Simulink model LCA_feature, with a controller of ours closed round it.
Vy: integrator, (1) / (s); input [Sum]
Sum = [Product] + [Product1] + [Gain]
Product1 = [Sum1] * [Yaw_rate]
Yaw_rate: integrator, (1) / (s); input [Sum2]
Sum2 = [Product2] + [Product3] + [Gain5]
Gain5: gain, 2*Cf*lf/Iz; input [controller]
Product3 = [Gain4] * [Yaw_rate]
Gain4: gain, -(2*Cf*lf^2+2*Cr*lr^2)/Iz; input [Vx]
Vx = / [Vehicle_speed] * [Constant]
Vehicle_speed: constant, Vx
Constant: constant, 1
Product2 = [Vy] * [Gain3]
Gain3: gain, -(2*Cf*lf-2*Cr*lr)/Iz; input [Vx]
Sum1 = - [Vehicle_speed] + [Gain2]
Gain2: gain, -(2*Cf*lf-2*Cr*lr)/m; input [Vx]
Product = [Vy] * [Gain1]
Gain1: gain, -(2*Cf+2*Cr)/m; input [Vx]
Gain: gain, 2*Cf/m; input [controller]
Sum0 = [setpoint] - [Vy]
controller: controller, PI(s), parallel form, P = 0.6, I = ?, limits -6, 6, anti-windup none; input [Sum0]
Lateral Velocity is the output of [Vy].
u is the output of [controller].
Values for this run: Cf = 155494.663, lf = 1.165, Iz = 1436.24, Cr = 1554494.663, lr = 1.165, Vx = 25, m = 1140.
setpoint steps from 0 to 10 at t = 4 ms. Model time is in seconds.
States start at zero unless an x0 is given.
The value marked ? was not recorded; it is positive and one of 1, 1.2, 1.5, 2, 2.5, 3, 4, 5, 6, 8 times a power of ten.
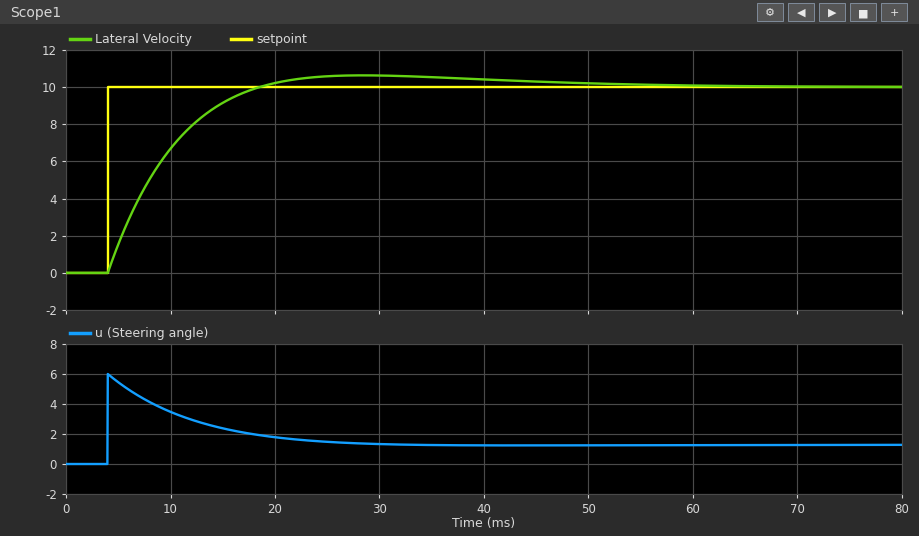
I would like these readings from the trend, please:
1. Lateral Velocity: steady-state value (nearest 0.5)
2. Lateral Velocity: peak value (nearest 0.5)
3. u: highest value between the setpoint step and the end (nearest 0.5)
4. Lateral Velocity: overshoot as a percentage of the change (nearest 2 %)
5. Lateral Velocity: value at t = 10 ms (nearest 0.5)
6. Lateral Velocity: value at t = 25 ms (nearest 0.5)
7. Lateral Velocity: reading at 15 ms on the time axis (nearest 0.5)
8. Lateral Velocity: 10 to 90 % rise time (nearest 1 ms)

10.0
10.5
6.0
6 %
6.5
10.5
9.0
10 ms
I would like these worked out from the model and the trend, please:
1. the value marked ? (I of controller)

40
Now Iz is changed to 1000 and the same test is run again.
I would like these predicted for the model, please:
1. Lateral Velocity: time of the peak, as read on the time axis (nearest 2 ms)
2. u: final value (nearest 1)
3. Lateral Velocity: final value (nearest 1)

26 ms
1
10
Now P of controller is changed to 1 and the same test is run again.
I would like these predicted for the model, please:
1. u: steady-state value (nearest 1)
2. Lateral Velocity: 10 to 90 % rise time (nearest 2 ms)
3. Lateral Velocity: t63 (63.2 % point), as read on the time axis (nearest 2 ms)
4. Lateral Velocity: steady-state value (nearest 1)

1
8 ms
8 ms
10
